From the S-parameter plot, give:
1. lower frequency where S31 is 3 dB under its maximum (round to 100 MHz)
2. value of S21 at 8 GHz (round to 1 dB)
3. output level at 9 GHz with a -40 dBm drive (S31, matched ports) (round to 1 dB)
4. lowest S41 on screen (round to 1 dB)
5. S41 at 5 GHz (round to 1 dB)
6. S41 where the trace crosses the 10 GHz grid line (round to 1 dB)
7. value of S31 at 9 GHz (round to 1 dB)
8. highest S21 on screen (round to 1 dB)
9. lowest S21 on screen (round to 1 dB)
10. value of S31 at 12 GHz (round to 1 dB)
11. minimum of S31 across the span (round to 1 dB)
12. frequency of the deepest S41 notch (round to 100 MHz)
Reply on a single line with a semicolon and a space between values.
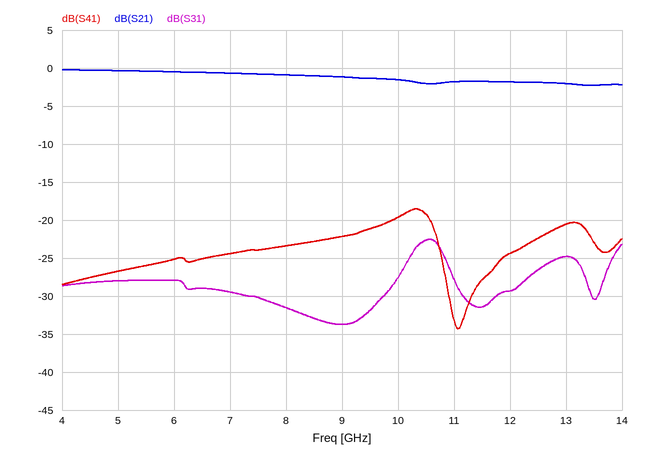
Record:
10.2 GHz; -1 dB; -74 dBm; -34 dB; -27 dB; -20 dB; -34 dB; 0 dB; -2 dB; -29 dB; -34 dB; 11.1 GHz
